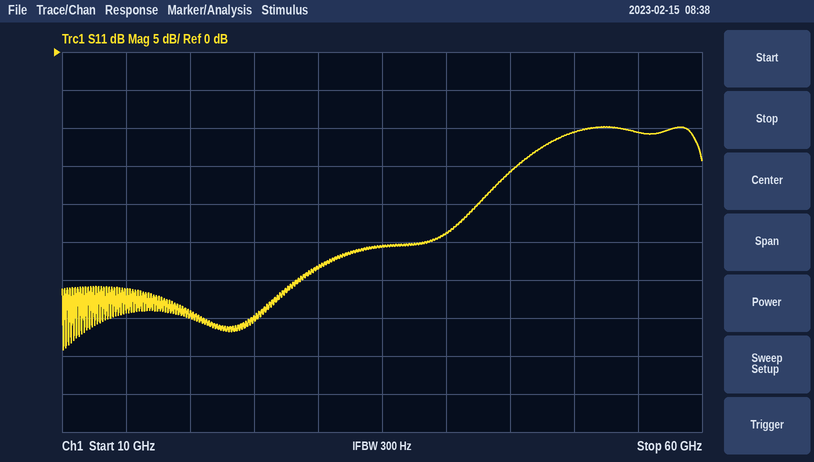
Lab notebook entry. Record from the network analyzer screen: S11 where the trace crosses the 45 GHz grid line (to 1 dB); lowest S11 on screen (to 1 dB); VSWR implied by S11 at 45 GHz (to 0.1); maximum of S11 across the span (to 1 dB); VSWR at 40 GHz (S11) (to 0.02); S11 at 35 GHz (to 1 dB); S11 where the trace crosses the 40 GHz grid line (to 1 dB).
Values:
-16 dB
-39 dB
1.4
-10 dB
1.14
-26 dB
-24 dB
